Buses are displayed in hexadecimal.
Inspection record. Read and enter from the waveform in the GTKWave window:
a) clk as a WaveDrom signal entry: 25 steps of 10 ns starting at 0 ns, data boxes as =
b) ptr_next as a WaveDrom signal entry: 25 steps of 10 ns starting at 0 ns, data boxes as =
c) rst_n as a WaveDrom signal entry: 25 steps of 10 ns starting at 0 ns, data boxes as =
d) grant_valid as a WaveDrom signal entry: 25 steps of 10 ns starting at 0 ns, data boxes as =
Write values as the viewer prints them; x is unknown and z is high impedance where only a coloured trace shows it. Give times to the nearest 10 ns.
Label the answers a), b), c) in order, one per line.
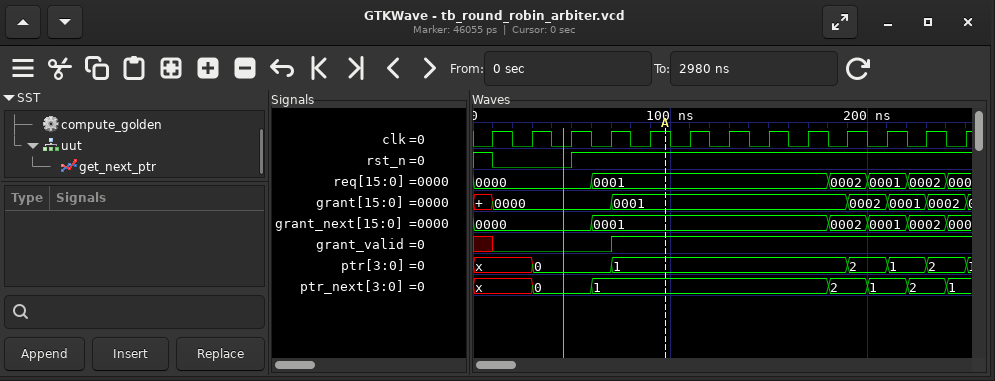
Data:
a) {name: 'clk', wave: '0101010101010101010101010'}
b) {name: 'ptr_next', wave: 'x..=..=...........=.=.=.=', data: '0 1 2 1 2 1'}
c) {name: 'rst_n', wave: '10...1...................'}
d) {name: 'grant_valid', wave: 'x0.....1.................'}
